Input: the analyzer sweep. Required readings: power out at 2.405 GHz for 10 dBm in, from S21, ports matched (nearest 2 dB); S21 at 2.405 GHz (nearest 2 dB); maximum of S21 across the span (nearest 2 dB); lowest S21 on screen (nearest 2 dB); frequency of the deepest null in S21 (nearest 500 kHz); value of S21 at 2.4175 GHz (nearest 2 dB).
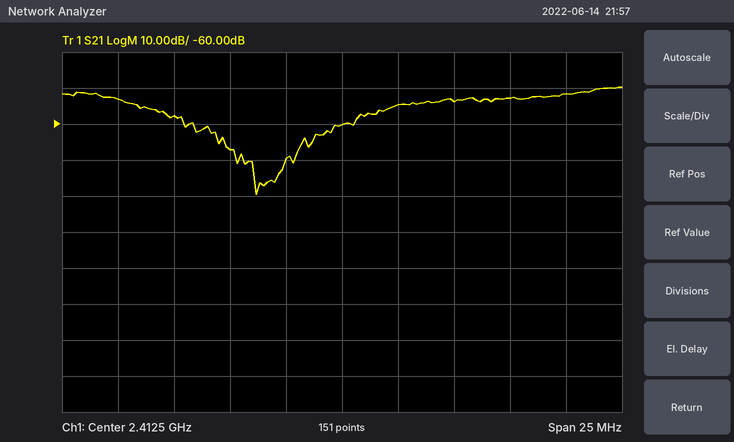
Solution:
-48 dBm
-58 dB
-50 dB
-80 dB
2.4085 GHz
-54 dB
